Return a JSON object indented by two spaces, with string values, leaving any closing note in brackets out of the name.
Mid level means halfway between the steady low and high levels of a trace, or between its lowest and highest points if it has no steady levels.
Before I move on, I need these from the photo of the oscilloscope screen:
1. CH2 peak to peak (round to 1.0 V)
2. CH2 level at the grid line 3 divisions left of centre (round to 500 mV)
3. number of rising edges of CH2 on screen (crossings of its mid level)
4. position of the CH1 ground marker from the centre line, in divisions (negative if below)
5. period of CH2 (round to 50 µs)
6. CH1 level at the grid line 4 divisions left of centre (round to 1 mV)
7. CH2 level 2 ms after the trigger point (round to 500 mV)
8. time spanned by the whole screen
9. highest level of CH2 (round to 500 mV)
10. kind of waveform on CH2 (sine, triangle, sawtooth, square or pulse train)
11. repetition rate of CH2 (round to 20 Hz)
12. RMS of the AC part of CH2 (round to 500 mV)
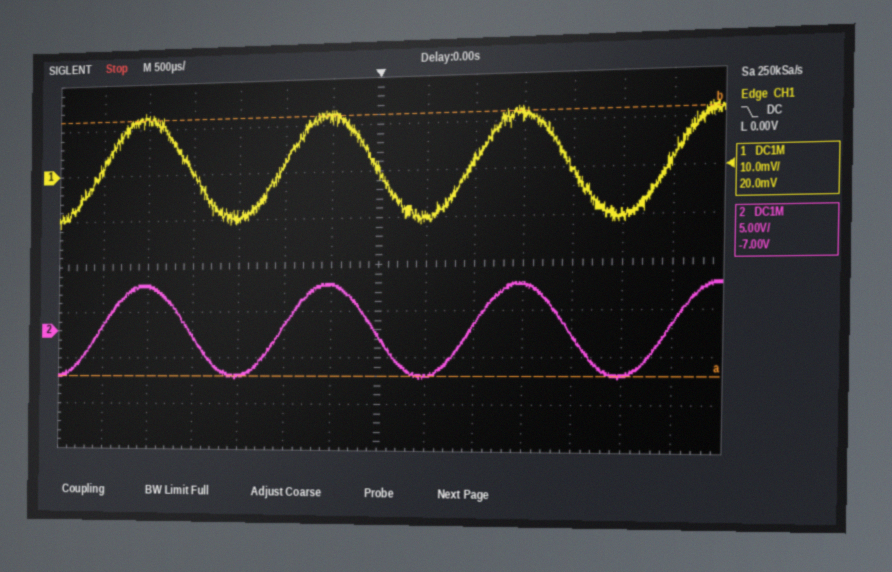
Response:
{
  "CH2 peak to peak": "10.0 V",
  "CH2 level at the grid line 3 divisions left of centre": "-5.0 V",
  "number of rising edges of CH2 on screen": "4",
  "position of the CH1 ground marker from the centre line, in divisions": "+2.0 div",
  "period of CH2": "2.00 ms",
  "CH1 level at the grid line 4 divisions left of centre": "0 mV",
  "CH2 level 2 ms after the trigger point": "-500 mV",
  "time spanned by the whole screen": "7 ms",
  "highest level of CH2": "5.0 V",
  "kind of waveform on CH2": "sine",
  "repetition rate of CH2": "500 Hz",
  "RMS of the AC part of CH2": "3.5 V"
}
